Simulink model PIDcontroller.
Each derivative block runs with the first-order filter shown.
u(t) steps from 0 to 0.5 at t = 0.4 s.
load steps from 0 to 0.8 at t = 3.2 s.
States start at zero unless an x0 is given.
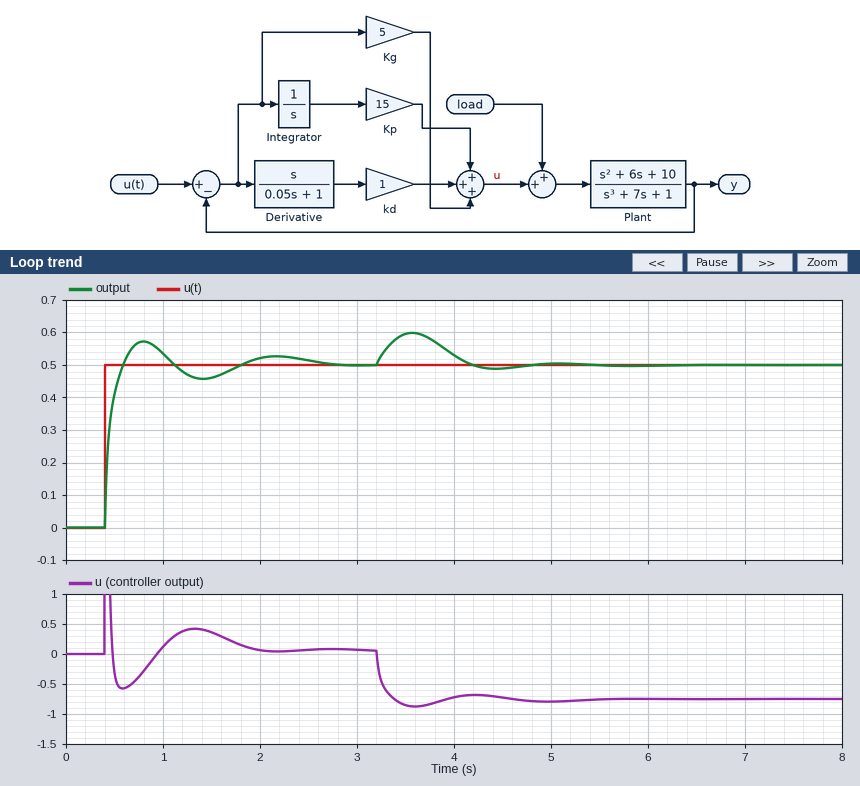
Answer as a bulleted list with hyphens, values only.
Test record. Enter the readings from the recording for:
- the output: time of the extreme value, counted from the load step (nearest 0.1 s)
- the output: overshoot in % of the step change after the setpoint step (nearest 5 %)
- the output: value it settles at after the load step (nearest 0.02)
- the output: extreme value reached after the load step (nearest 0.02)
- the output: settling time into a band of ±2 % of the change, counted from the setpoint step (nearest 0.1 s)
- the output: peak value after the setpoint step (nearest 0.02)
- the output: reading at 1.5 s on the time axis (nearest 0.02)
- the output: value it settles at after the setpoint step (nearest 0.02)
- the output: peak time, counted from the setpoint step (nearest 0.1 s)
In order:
- 0.4 s
- 15 %
- 0.50
- 0.60
- 2.2 s
- 0.58
- 0.46
- 0.50
- 0.4 s
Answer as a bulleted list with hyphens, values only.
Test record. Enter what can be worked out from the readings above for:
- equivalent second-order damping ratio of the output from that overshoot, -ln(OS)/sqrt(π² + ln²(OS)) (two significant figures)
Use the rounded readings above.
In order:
- 0.52
